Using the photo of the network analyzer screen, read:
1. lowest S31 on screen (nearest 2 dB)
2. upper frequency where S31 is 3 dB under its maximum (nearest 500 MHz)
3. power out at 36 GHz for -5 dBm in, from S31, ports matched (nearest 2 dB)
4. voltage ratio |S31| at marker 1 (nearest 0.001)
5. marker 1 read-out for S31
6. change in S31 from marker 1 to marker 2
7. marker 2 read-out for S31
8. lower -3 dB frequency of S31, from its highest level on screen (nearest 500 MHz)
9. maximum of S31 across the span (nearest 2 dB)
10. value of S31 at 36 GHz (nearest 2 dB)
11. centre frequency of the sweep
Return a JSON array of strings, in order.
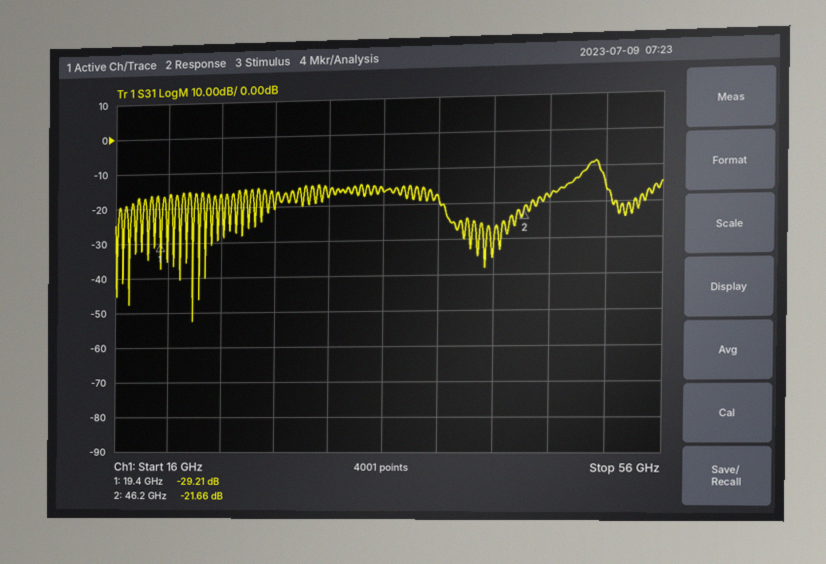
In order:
["-52 dB", "51.5 GHz", "-22 dBm", "0.035", "-29.21 dB", "7.55 dB", "-21.66 dB", "50.5 GHz", "-8 dB", "-16 dB", "36 GHz"]
